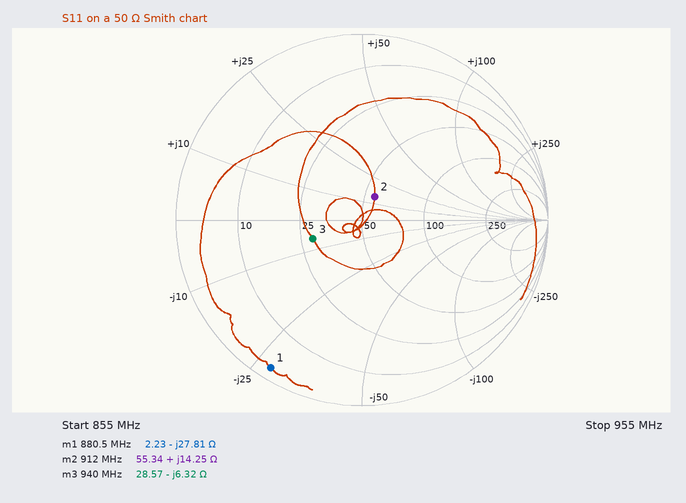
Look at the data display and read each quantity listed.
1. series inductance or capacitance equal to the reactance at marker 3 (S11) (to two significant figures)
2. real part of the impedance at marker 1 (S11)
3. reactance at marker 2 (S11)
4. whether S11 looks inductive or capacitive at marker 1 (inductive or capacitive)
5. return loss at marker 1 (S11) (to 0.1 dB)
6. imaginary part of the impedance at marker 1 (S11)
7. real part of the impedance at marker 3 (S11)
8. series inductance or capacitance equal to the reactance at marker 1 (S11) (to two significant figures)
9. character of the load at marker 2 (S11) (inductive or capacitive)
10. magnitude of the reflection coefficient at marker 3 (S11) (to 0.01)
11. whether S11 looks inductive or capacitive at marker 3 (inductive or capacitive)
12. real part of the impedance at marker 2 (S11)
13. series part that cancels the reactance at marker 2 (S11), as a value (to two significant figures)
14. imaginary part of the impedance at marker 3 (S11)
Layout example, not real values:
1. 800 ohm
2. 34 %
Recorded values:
1. 27 pF
2. 2.23 Ω
3. +14.25 Ω
4. capacitive
5. 0.6 dB
6. -27.81 Ω
7. 28.57 Ω
8. 6.5 pF
9. inductive
10. 0.28
11. capacitive
12. 55.34 Ω
13. 12 pF
14. -6.32 Ω
